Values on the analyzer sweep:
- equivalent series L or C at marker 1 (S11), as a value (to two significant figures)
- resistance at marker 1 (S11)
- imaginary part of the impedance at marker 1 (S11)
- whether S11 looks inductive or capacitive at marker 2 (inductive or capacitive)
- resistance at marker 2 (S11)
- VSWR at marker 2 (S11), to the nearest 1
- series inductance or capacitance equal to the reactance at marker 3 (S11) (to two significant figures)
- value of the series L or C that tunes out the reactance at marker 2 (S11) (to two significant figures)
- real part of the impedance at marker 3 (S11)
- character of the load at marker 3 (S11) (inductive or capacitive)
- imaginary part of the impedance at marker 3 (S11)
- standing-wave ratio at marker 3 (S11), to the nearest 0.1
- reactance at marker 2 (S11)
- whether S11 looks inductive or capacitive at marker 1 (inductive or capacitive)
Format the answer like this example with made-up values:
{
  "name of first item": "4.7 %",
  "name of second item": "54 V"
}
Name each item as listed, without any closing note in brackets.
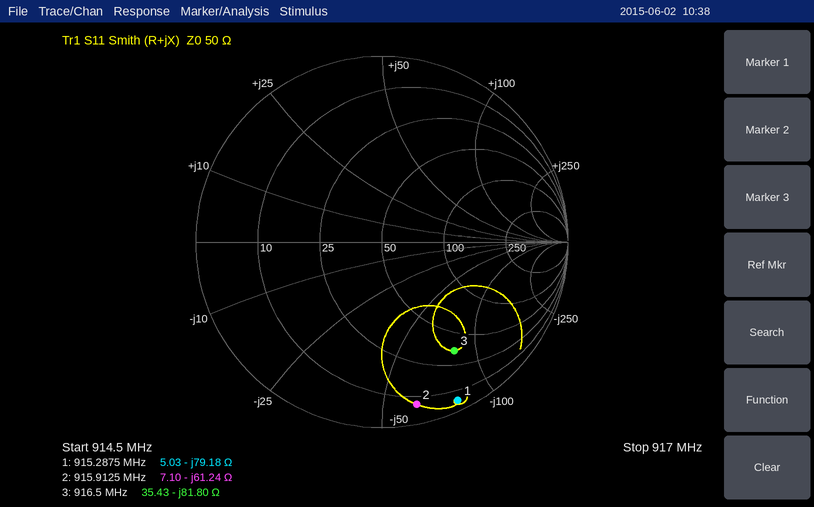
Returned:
{
  "equivalent series L or C at marker 1 (S11), as a value": "2.2 pF",
  "resistance at marker 1": "5.03 Ω",
  "imaginary part of the impedance at marker 1": "-79.18 Ω",
  "whether S11 looks inductive or capacitive at marker 2": "capacitive",
  "resistance at marker 2": "7.10 Ω",
  "VSWR at marker 2 (S11), to the nearest 1": "18",
  "series inductance or capacitance equal to the reactance at marker 3 (S11)": "2.1 pF",
  "value of the series L or C that tunes out the reactance at marker 2 (S11)": "11 nH",
  "real part of the impedance at marker 3": "35.43 Ω",
  "character of the load at marker 3 (S11)": "capacitive",
  "imaginary part of the impedance at marker 3": "-81.80 Ω",
  "standing-wave ratio at marker 3 (S11), to the nearest 0.1": "5.7",
  "reactance at marker 2": "-61.24 Ω",
  "whether S11 looks inductive or capacitive at marker 1": "capacitive"
}
